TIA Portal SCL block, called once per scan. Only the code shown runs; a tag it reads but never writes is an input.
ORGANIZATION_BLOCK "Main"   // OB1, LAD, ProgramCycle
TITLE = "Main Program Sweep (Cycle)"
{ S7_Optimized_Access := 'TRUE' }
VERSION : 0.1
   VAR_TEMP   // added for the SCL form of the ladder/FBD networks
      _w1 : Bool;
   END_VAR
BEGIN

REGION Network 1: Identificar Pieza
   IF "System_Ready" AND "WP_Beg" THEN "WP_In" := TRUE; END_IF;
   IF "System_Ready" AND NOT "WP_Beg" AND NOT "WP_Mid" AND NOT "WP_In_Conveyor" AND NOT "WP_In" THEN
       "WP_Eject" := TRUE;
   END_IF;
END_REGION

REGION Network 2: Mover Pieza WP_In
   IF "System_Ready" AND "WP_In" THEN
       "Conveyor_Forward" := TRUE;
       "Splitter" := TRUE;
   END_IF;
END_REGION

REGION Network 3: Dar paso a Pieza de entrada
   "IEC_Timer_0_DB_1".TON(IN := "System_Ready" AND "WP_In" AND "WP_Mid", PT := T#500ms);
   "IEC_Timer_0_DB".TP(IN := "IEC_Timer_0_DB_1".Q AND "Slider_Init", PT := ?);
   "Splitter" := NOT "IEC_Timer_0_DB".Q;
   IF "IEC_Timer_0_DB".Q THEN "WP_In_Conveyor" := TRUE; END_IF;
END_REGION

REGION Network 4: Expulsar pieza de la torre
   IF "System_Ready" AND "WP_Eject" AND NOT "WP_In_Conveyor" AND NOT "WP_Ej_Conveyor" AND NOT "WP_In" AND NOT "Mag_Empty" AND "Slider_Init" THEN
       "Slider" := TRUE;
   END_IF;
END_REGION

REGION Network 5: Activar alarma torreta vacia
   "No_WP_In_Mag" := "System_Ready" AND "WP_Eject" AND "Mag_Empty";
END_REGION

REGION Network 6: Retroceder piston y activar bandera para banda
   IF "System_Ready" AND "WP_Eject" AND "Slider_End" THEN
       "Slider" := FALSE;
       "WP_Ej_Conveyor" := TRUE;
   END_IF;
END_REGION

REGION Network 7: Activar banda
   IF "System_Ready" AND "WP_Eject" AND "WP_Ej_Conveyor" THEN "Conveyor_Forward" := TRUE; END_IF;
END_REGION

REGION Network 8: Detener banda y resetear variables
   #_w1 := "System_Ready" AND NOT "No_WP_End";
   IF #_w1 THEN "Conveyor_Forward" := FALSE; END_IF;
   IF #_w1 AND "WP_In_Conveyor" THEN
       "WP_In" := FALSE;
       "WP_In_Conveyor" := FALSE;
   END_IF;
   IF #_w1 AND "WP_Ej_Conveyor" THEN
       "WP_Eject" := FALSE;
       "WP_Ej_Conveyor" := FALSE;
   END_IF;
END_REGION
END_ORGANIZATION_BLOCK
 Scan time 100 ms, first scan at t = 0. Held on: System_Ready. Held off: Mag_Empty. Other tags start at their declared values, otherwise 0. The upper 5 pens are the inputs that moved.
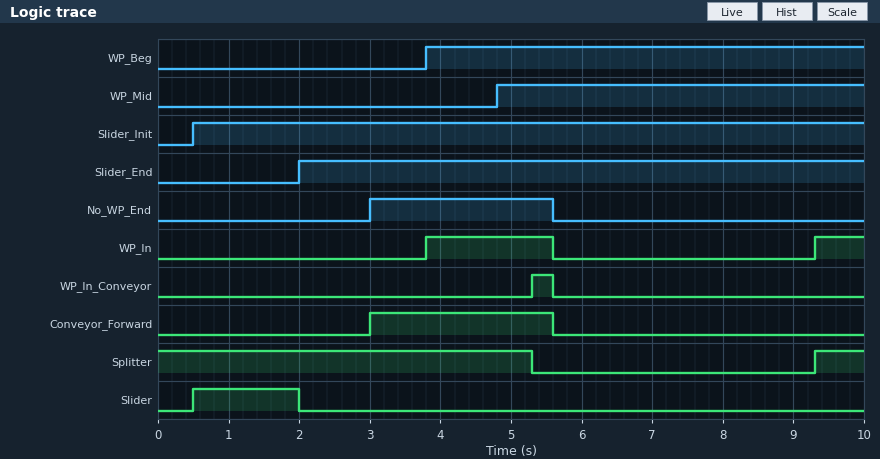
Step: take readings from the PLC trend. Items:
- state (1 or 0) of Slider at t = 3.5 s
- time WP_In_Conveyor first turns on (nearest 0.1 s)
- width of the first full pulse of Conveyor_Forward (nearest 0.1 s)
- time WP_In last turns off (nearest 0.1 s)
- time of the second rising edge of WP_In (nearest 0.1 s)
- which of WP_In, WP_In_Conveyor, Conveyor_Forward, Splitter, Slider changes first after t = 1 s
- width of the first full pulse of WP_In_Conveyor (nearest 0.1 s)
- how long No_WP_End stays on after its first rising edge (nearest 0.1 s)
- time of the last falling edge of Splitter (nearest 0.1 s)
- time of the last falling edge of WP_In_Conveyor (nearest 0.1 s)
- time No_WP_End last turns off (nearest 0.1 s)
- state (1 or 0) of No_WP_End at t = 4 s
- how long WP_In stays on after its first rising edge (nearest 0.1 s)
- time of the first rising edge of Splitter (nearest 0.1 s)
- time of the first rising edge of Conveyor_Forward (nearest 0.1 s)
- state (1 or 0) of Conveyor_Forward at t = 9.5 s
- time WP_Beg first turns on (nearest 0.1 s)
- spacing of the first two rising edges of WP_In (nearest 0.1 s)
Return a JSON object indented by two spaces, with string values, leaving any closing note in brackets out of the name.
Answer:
{
  "state (1 or 0) of Slider at t = 3.5 s": "0",
  "time WP_In_Conveyor first turns on": "5.3 s",
  "width of the first full pulse of Conveyor_Forward": "2.6 s",
  "time WP_In last turns off": "5.6 s",
  "time of the second rising edge of WP_In": "9.3 s",
  "which of WP_In, WP_In_Conveyor, Conveyor_Forward, Splitter, Slider changes first after t = 1 s": "Slider",
  "width of the first full pulse of WP_In_Conveyor": "0.3 s",
  "how long No_WP_End stays on after its first rising edge": "2.6 s",
  "time of the last falling edge of Splitter": "5.3 s",
  "time of the last falling edge of WP_In_Conveyor": "5.6 s",
  "time No_WP_End last turns off": "5.6 s",
  "state (1 or 0) of No_WP_End at t = 4 s": "1",
  "how long WP_In stays on after its first rising edge": "1.8 s",
  "time of the first rising edge of Splitter": "9.3 s",
  "time of the first rising edge of Conveyor_Forward": "3.0 s",
  "state (1 or 0) of Conveyor_Forward at t = 9.5 s": "0",
  "time WP_Beg first turns on": "3.8 s",
  "spacing of the first two rising edges of WP_In": "5.5 s"
}
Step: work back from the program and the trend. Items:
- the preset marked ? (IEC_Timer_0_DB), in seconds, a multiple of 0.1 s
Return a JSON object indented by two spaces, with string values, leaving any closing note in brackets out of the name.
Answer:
{
  "the preset marked ? (IEC_Timer_0_DB), in seconds, a multiple of 0.1 s": "4.0 s"
}
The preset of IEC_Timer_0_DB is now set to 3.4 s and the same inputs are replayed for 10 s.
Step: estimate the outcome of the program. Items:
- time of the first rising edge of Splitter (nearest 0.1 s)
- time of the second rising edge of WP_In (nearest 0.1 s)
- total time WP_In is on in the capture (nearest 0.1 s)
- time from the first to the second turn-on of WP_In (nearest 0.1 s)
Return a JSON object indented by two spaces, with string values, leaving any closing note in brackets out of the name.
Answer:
{
  "time of the first rising edge of Splitter": "8.7 s",
  "time of the second rising edge of WP_In": "8.7 s",
  "total time WP_In is on in the capture": "3.1 s",
  "time from the first to the second turn-on of WP_In": "4.9 s"
}
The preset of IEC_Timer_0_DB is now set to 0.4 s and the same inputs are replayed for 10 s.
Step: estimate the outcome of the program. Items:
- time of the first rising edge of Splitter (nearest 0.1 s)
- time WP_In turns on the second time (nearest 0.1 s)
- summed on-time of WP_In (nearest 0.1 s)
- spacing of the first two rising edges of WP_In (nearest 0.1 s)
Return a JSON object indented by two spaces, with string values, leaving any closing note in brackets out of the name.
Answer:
{
  "time of the first rising edge of Splitter": "5.7 s",
  "time WP_In turns on the second time": "5.7 s",
  "summed on-time of WP_In": "6.1 s",
  "spacing of the first two rising edges of WP_In": "1.9 s"
}
